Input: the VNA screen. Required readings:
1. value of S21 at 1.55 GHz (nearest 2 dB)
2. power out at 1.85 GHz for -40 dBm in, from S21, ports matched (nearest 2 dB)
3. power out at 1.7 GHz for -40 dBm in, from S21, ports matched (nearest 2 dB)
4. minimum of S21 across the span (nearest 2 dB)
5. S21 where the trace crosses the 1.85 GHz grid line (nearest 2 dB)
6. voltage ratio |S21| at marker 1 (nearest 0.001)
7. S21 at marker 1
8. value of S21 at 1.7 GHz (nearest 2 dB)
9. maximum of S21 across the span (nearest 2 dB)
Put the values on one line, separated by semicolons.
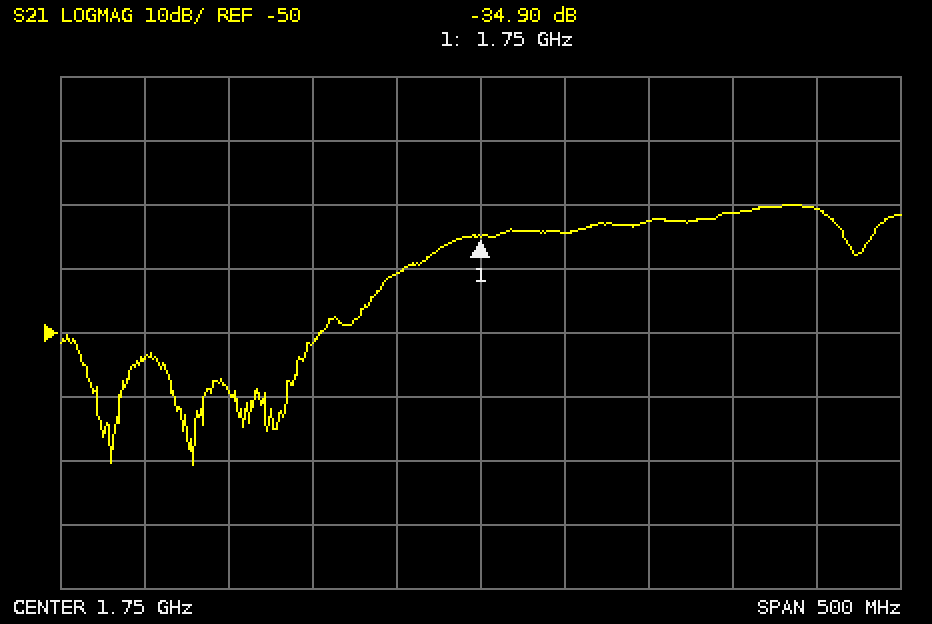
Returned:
-54 dB; -72 dBm; -80 dBm; -70 dB; -32 dB; 0.018; -34.90 dB; -40 dB; -30 dB
